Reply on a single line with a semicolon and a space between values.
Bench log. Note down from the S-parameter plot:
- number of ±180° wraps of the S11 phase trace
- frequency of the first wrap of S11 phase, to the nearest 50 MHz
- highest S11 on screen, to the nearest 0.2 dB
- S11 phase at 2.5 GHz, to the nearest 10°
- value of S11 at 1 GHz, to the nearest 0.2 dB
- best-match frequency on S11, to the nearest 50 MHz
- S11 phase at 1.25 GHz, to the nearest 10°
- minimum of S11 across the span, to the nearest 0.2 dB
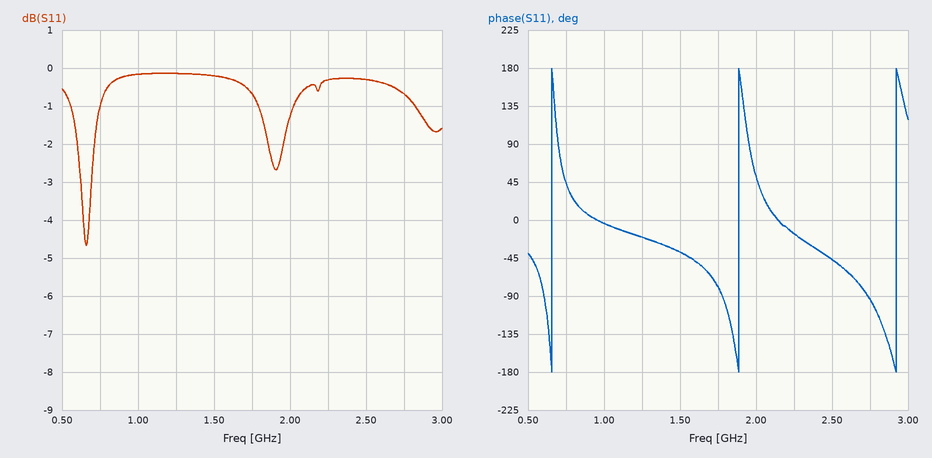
3; 650 MHz; -0.2 dB; -50°; -0.2 dB; 650 MHz; -20°; -4.6 dB
